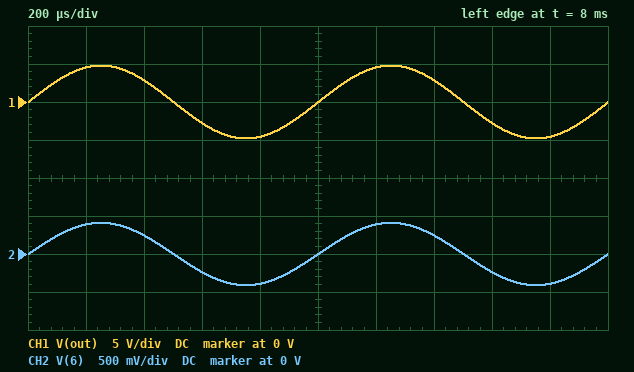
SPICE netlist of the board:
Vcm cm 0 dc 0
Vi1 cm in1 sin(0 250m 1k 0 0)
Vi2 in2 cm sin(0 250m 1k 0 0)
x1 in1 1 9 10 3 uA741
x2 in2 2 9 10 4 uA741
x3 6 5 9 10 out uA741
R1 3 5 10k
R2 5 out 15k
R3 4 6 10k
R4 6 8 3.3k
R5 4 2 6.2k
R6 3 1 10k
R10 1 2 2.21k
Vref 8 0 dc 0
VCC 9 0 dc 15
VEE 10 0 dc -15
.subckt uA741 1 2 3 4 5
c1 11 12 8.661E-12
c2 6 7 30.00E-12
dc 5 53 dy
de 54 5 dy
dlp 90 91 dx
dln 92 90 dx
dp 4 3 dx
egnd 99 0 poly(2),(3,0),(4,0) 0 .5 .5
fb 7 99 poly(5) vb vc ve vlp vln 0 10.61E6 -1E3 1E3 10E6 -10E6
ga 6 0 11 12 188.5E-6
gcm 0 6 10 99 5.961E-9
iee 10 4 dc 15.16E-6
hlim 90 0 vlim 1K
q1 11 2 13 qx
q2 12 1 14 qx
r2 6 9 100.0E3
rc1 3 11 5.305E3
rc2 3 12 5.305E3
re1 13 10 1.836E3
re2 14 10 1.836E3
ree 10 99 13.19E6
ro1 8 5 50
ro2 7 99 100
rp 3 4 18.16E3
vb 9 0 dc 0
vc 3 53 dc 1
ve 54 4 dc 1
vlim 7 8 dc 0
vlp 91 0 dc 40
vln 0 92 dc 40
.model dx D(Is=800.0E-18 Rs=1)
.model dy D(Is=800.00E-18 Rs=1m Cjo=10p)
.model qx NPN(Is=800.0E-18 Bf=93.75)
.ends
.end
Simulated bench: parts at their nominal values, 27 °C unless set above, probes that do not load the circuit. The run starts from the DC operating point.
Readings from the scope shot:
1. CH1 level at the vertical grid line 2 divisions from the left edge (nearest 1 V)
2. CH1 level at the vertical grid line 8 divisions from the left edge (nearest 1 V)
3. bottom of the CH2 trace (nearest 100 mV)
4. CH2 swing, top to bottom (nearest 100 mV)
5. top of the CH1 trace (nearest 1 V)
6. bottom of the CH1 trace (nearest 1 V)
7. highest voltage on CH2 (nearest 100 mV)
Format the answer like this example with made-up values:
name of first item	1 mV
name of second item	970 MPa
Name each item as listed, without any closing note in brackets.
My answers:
CH1 level at the vertical grid line 2 divisions from the left edge	3 V
CH1 level at the vertical grid line 8 divisions from the left edge	-3 V
bottom of the CH2 trace	-400 mV
CH2 swing, top to bottom	800 mV
top of the CH1 trace	5 V
bottom of the CH1 trace	-5 V
highest voltage on CH2	400 mV
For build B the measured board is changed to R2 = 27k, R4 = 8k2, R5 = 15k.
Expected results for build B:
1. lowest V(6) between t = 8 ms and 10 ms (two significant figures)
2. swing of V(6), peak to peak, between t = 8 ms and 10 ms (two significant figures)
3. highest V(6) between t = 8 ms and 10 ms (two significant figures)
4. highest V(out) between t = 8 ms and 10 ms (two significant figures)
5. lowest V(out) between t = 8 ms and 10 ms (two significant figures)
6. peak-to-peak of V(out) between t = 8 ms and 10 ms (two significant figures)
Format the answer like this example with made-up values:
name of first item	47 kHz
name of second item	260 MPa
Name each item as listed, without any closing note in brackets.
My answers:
lowest V(6) between t = 8 ms and 10 ms	-1.6 V
swing of V(6), peak to peak, between t = 8 ms and 10 ms	3.3 V
highest V(6) between t = 8 ms and 10 ms	1.6 V
highest V(out) between t = 8 ms and 10 ms	13 V
lowest V(out) between t = 8 ms and 10 ms	-13 V
peak-to-peak of V(out) between t = 8 ms and 10 ms	26 V
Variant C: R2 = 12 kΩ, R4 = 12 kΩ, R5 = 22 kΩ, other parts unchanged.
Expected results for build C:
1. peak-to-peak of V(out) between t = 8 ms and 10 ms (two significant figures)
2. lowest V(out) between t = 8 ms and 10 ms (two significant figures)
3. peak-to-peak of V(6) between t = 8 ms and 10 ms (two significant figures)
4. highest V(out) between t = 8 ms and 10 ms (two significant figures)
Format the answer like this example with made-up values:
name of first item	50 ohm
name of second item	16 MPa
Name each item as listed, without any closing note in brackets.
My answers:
peak-to-peak of V(out) between t = 8 ms and 10 ms	19 V
lowest V(out) between t = 8 ms and 10 ms	-9.3 V
peak-to-peak of V(6) between t = 8 ms and 10 ms	5.7 V
highest V(out) between t = 8 ms and 10 ms	9.3 V
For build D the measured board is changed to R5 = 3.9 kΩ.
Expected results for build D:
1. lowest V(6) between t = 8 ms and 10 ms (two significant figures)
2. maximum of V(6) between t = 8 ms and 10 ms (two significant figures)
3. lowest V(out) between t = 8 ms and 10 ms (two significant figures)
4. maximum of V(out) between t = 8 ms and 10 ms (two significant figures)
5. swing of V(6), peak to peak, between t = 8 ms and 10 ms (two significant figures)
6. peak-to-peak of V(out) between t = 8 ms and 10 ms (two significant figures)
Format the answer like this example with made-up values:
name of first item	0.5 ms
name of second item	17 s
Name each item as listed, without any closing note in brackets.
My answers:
lowest V(6) between t = 8 ms and 10 ms	-280 mV
maximum of V(6) between t = 8 ms and 10 ms	280 mV
lowest V(out) between t = 8 ms and 10 ms	-4.5 V
maximum of V(out) between t = 8 ms and 10 ms	4.5 V
swing of V(6), peak to peak, between t = 8 ms and 10 ms	560 mV
peak-to-peak of V(out) between t = 8 ms and 10 ms	8.9 V
